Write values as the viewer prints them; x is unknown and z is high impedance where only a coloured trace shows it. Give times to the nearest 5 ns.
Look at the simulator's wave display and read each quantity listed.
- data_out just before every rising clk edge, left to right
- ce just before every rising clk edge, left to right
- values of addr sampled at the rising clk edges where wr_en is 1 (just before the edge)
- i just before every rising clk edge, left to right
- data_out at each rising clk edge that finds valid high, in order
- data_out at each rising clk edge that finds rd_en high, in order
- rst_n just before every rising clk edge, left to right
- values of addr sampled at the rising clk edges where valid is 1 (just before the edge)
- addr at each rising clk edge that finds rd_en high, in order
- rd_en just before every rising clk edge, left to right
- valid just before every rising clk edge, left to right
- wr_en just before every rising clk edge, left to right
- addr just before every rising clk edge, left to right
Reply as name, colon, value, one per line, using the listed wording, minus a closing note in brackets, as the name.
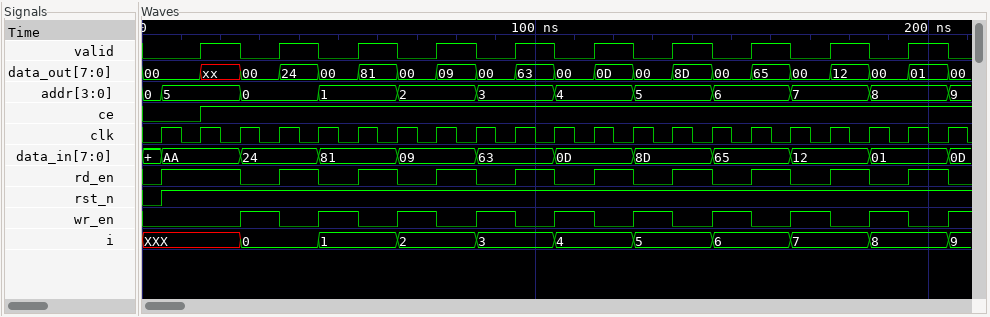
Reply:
data_out just before every rising clk edge, left to right: 00, 00, xx, 00, 24, 00, 81, 00, 09, 00, 63, 00, 0D, 00, 8D, 00, 65, 00, 12, 00, 01
ce just before every rising clk edge, left to right: 0 0 1 1 1 1 1 1 1 1 1 1 1 1 1 1 1 1 1 1 1
values of addr sampled at the rising clk edges where wr_en is 1: 0, 1, 2, 3, 4, 5, 6, 7, 8
i just before every rising clk edge, left to right: XXX, XXX, XXX, 0, 0, 1, 1, 2, 2, 3, 3, 4, 4, 5, 5, 6, 6, 7, 7, 8, 8
data_out at each rising clk edge that finds valid high, in order: xx, 24, 81, 09, 63, 0D, 8D, 65, 12, 01
data_out at each rising clk edge that finds rd_en high, in order: 00, xx, 24, 81, 09, 63, 0D, 8D, 65, 12, 01
rst_n just before every rising clk edge, left to right: 0 1 1 1 1 1 1 1 1 1 1 1 1 1 1 1 1 1 1 1 1
values of addr sampled at the rising clk edges where valid is 1: 5, 0, 1, 2, 3, 4, 5, 6, 7, 8
addr at each rising clk edge that finds rd_en high, in order: 5, 5, 0, 1, 2, 3, 4, 5, 6, 7, 8
rd_en just before every rising clk edge, left to right: 0 1 1 0 1 0 1 0 1 0 1 0 1 0 1 0 1 0 1 0 1
valid just before every rising clk edge, left to right: 0 0 1 0 1 0 1 0 1 0 1 0 1 0 1 0 1 0 1 0 1
wr_en just before every rising clk edge, left to right: 0 0 0 1 0 1 0 1 0 1 0 1 0 1 0 1 0 1 0 1 0
addr just before every rising clk edge, left to right: 0, 5, 5, 0, 0, 1, 1, 2, 2, 3, 3, 4, 4, 5, 5, 6, 6, 7, 7, 8, 8
